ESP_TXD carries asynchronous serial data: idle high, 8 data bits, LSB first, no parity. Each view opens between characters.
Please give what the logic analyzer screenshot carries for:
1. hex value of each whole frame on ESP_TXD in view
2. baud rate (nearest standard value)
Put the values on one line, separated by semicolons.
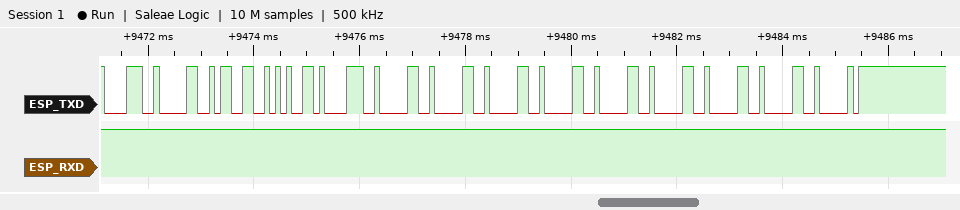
38, 30, 33, 65, 38, 30, 30, 30, 30, 30, 30, 30, 30, D0; 9600 baud
